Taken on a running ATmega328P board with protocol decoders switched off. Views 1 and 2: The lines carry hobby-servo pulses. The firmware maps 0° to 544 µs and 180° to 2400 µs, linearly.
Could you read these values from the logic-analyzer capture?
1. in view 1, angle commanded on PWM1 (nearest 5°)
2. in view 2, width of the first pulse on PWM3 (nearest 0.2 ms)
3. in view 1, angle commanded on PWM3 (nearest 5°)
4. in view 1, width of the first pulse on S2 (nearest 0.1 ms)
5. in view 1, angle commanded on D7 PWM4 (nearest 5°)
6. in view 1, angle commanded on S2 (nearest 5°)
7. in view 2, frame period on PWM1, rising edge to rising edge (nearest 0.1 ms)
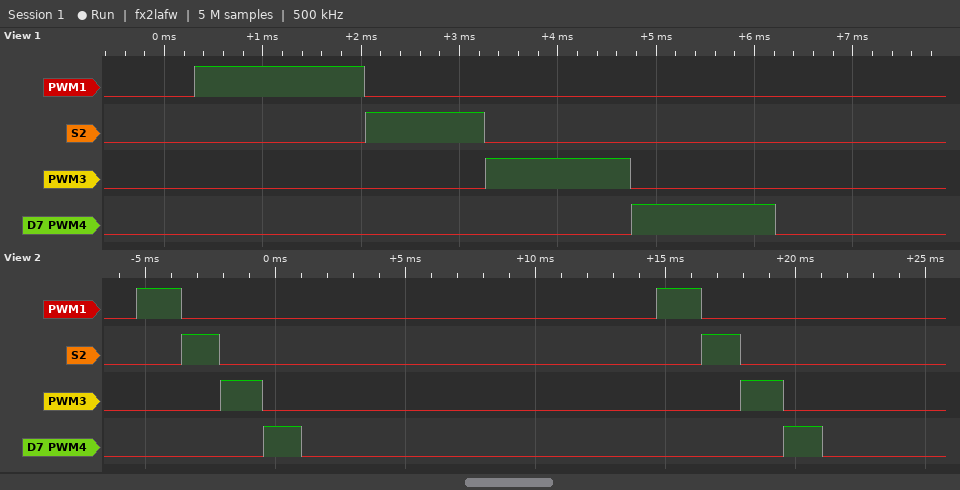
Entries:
115°
1.6 ms
90°
1.2 ms
90°
65°
20.0 ms
